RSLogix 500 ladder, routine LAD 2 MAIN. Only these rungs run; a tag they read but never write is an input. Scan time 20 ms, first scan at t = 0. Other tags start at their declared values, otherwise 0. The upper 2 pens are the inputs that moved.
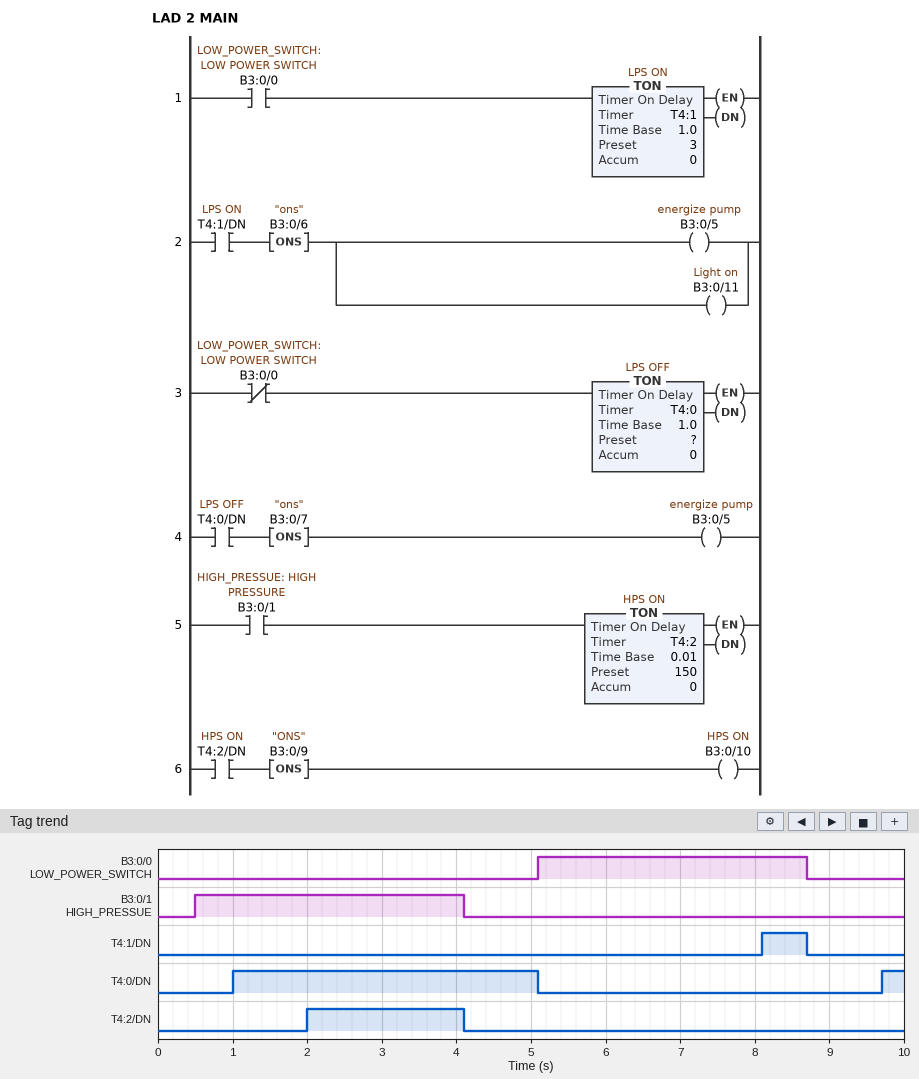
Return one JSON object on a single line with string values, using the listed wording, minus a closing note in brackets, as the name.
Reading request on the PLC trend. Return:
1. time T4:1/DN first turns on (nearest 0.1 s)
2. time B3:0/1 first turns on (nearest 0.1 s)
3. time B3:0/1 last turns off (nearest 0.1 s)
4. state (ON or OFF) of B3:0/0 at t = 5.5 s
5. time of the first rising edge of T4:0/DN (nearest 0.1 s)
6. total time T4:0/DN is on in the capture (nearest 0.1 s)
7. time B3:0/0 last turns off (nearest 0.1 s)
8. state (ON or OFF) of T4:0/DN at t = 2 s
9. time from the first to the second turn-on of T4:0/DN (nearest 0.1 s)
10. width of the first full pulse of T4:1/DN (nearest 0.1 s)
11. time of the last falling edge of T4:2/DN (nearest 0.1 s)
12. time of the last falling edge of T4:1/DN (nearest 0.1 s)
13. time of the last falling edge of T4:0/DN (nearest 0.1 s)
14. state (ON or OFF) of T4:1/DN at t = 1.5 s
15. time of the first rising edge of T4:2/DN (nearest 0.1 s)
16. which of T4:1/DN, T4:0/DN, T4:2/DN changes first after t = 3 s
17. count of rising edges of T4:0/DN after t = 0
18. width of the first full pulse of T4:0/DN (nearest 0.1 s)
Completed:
{"time T4:1/DN first turns on": "8.1 s", "time B3:0/1 first turns on": "0.5 s", "time B3:0/1 last turns off": "4.1 s", "state (ON or OFF) of B3:0/0 at t = 5.5 s": "ON", "time of the first rising edge of T4:0/DN": "1.0 s", "total time T4:0/DN is on in the capture": "4.4 s", "time B3:0/0 last turns off": "8.7 s", "state (ON or OFF) of T4:0/DN at t = 2 s": "ON", "time from the first to the second turn-on of T4:0/DN": "8.7 s", "width of the first full pulse of T4:1/DN": "0.6 s", "time of the last falling edge of T4:2/DN": "4.1 s", "time of the last falling edge of T4:1/DN": "8.7 s", "time of the last falling edge of T4:0/DN": "5.1 s", "state (ON or OFF) of T4:1/DN at t = 1.5 s": "OFF", "time of the first rising edge of T4:2/DN": "2.0 s", "which of T4:1/DN, T4:0/DN, T4:2/DN changes first after t = 3 s": "T4:2/DN", "count of rising edges of T4:0/DN after t = 0": "2", "width of the first full pulse of T4:0/DN": "4.1 s"}
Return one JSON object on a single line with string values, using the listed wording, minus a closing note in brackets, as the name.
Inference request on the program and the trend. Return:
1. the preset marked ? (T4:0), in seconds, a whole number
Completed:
{"the preset marked ? (T4:0), in seconds, a whole number": "1 s"}
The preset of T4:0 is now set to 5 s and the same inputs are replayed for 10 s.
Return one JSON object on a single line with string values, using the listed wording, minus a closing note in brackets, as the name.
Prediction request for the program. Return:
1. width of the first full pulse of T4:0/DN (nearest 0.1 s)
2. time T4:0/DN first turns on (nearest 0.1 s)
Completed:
{"width of the first full pulse of T4:0/DN": "0.1 s", "time T4:0/DN first turns on": "5.0 s"}
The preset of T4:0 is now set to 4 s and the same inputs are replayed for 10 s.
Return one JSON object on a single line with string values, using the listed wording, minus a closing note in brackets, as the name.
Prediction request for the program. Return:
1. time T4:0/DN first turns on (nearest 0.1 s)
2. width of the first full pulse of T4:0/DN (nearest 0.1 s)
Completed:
{"time T4:0/DN first turns on": "4.0 s", "width of the first full pulse of T4:0/DN": "1.1 s"}
